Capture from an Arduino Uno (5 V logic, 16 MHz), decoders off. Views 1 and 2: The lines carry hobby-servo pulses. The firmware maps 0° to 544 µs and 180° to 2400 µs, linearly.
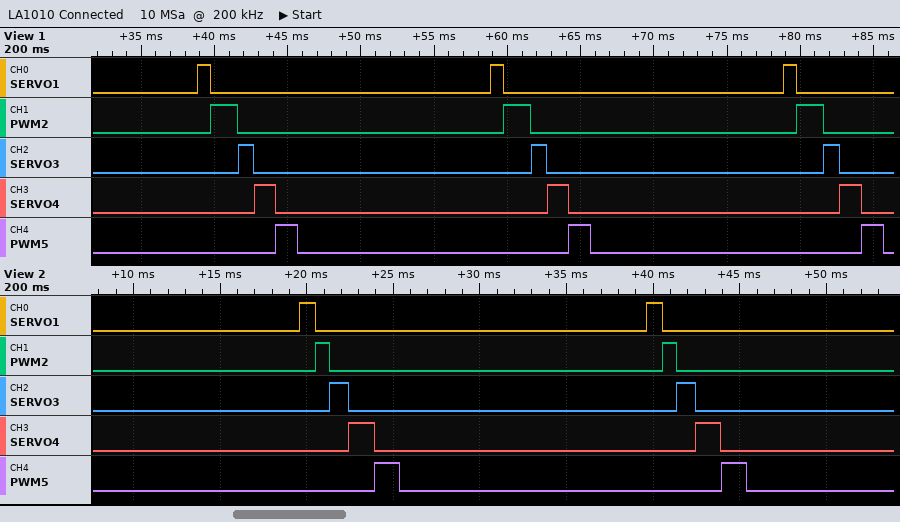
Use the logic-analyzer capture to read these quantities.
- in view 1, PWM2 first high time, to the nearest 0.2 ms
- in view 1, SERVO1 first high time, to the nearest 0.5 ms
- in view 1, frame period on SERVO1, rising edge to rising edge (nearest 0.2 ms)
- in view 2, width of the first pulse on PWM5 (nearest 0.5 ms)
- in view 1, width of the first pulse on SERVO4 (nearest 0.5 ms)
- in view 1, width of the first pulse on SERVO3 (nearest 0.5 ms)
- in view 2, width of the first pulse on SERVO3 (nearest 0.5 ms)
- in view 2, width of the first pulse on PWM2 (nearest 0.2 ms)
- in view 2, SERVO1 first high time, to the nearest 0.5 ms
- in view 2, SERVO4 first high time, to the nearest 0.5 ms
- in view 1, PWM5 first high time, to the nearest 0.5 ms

1.8 ms
1.0 ms
20.0 ms
1.5 ms
1.5 ms
1.0 ms
1.0 ms
0.8 ms
1.0 ms
1.5 ms
1.5 ms
